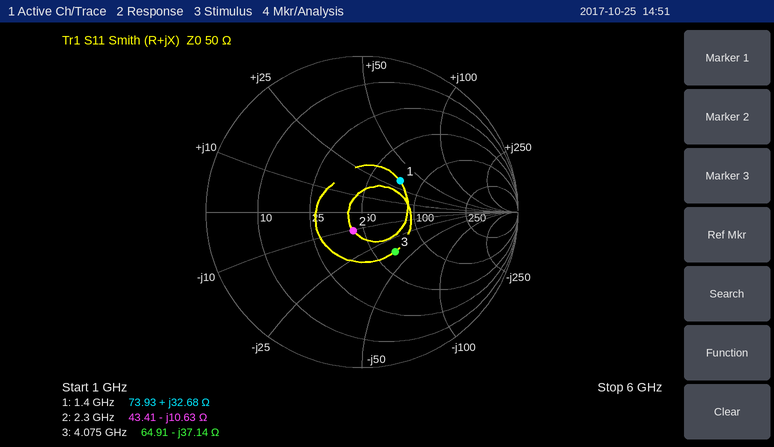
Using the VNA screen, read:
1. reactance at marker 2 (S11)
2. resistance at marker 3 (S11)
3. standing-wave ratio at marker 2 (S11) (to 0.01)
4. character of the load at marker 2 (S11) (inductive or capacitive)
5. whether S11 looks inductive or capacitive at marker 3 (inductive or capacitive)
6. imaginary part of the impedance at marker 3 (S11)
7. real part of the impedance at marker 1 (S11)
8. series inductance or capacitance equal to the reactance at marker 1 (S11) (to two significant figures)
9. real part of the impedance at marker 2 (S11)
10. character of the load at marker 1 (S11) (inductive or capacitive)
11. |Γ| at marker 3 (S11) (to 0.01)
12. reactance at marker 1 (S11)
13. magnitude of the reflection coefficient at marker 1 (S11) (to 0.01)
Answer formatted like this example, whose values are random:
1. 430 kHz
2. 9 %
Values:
1. -10.63 Ω
2. 64.91 Ω
3. 1.31
4. capacitive
5. capacitive
6. -37.14 Ω
7. 73.93 Ω
8. 3.7 nH
9. 43.41 Ω
10. inductive
11. 0.33
12. +32.68 Ω
13. 0.32
